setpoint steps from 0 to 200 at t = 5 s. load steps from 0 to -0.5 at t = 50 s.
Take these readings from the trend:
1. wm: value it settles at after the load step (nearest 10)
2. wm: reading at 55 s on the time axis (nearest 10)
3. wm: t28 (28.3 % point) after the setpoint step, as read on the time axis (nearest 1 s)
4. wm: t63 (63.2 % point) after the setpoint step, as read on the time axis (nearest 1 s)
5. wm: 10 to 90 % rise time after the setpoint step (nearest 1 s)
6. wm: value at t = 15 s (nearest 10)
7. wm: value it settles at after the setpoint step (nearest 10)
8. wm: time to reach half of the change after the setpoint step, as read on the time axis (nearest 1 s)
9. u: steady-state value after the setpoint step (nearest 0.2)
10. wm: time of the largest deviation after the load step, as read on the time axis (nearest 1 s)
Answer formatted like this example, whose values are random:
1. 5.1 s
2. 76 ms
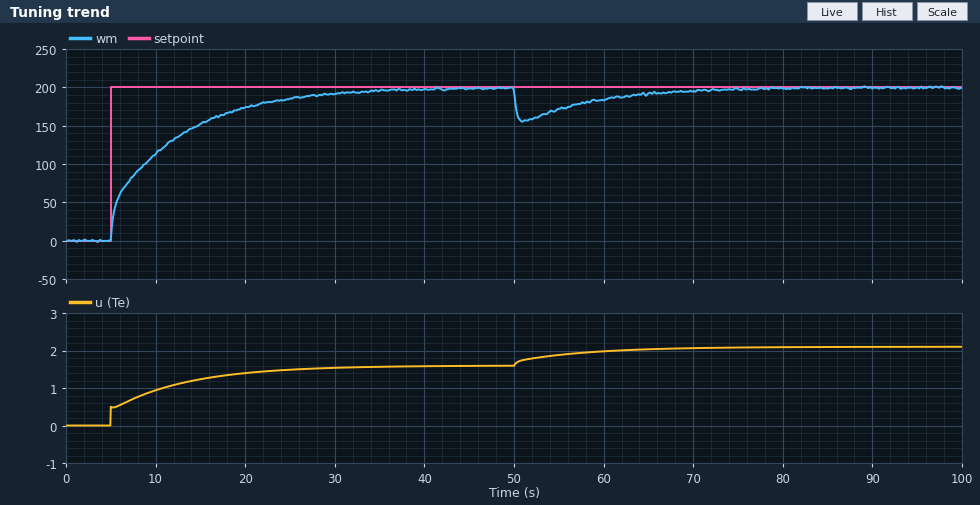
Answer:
1. 200
2. 170
3. 6 s
4. 11 s
5. 17 s
6. 150
7. 200
8. 9 s
9. 1.6
10. 51 s
